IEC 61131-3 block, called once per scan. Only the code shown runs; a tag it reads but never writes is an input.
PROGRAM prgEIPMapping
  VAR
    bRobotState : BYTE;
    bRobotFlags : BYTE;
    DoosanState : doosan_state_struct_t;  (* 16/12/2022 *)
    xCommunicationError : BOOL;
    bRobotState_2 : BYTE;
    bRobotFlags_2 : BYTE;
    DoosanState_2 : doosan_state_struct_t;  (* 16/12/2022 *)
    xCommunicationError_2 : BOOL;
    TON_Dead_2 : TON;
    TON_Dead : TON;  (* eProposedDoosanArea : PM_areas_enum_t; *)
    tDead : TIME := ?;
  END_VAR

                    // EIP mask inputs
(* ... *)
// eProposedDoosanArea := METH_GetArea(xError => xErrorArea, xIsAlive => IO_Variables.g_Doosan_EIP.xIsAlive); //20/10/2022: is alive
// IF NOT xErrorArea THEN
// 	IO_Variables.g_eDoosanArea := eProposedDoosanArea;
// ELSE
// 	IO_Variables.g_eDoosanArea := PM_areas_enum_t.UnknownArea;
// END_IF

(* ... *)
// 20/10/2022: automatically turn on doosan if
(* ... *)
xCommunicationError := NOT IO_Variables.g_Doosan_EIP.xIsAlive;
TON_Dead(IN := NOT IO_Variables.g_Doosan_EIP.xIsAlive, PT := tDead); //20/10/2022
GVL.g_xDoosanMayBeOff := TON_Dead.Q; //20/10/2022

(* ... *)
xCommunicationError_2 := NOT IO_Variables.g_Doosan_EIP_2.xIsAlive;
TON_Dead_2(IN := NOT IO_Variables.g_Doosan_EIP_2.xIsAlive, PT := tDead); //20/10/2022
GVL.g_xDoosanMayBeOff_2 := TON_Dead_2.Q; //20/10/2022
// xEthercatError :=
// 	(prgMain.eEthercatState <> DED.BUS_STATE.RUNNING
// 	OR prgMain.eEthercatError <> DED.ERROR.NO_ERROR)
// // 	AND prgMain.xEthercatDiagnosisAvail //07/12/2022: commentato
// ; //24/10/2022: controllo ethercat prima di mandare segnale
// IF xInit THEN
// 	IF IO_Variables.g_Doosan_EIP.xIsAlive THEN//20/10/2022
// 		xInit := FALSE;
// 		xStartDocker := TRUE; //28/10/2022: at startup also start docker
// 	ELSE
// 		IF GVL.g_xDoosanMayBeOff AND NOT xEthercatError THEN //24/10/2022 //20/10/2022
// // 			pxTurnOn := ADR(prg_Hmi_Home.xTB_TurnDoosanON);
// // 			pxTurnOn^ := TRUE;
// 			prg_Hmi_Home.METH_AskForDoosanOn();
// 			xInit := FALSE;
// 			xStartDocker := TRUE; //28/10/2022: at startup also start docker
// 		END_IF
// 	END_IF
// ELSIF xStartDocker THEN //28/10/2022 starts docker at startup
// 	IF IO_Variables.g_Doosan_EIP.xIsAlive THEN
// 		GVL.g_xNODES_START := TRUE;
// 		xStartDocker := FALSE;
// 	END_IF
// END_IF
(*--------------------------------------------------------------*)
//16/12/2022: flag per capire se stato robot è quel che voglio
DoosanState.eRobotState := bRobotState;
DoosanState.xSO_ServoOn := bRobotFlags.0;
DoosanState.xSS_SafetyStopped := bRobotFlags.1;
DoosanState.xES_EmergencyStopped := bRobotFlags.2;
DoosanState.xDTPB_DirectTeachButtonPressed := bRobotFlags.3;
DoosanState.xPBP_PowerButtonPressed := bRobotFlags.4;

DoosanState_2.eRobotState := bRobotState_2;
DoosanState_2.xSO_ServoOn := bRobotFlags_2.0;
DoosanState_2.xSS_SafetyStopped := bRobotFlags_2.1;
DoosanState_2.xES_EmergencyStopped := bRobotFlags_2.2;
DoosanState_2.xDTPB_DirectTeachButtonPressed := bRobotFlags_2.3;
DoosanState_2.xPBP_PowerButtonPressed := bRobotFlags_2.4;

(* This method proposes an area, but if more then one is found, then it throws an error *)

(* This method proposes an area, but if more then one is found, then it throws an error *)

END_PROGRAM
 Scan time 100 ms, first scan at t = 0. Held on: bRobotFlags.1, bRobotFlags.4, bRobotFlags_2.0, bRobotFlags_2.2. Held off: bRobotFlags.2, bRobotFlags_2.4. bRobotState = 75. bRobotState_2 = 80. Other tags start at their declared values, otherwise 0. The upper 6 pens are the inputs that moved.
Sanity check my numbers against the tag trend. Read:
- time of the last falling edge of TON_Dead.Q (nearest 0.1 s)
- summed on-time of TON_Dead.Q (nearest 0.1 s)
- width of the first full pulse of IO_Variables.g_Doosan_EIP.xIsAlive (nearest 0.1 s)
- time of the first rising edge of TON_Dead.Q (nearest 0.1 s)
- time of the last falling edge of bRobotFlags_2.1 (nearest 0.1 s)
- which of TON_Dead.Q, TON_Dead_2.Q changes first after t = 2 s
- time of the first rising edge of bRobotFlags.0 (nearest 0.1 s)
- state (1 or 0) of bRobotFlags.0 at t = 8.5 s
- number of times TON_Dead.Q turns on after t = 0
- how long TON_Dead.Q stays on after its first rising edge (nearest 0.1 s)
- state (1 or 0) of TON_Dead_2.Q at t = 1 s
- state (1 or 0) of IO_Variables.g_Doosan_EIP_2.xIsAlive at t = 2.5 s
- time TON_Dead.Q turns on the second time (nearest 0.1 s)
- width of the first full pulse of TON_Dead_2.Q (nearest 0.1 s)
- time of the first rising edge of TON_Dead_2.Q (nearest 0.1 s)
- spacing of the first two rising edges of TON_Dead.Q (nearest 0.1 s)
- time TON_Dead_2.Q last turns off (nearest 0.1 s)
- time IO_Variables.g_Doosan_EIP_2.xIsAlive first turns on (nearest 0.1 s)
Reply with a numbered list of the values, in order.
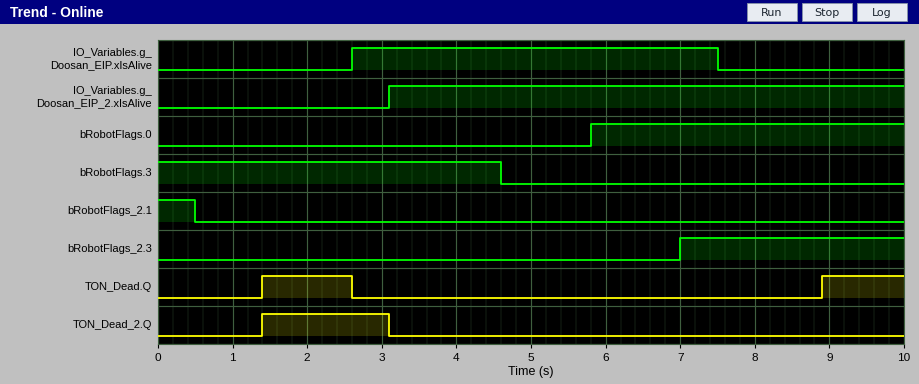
1. 2.6 s
2. 2.3 s
3. 4.9 s
4. 1.4 s
5. 0.5 s
6. TON_Dead.Q
7. 5.8 s
8. 1
9. 2
10. 1.2 s
11. 0
12. 0
13. 8.9 s
14. 1.7 s
15. 1.4 s
16. 7.5 s
17. 3.1 s
18. 3.1 s
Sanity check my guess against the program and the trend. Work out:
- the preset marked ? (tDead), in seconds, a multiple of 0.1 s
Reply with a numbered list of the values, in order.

1. 1.4 s
